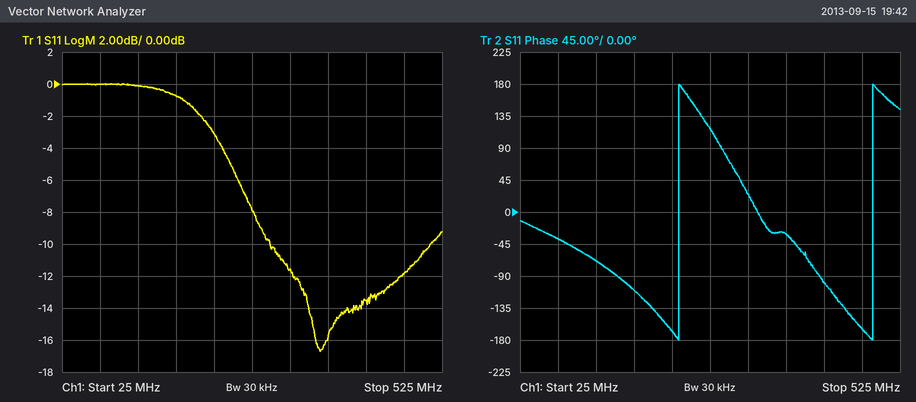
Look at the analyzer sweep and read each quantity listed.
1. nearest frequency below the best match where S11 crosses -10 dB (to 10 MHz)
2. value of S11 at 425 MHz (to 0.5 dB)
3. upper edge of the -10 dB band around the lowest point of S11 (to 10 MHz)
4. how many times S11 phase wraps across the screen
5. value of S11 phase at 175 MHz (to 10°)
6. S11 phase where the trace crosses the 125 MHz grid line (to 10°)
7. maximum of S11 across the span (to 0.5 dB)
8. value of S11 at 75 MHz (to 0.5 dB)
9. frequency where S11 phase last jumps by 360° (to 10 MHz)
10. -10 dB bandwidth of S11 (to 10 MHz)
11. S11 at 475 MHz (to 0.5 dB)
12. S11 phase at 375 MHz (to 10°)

300 MHz
-13.5 dB
510 MHz
2
-110°
-70°
0.0 dB
0.0 dB
490 MHz
210 MHz
-12.0 dB
-30°
